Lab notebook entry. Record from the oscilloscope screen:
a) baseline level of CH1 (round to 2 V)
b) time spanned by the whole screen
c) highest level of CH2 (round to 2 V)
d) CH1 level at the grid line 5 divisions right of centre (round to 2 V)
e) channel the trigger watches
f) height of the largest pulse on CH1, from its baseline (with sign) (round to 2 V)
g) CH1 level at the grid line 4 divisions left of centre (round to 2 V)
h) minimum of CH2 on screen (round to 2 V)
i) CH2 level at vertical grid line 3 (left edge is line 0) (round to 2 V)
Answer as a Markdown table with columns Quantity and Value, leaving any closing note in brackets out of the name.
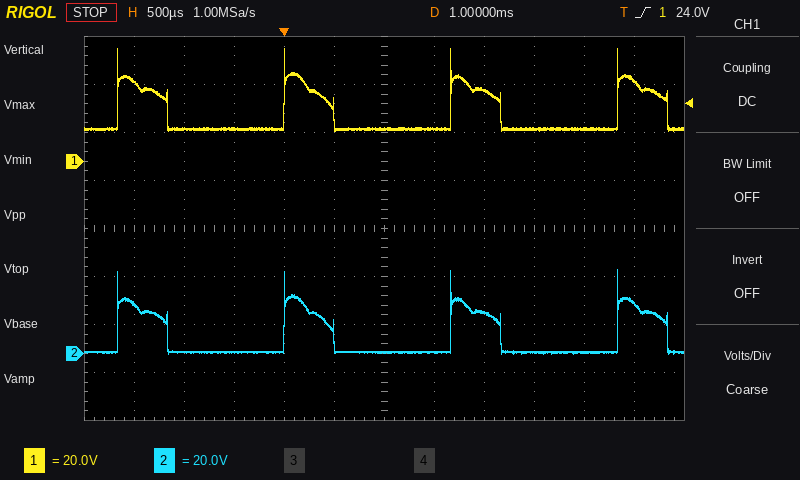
| Quantity | Value |
|---|---|
| baseline level of CH1 | 14 V |
| time spanned by the whole screen | 6 ms |
| highest level of CH2 | 34 V |
| CH1 level at the grid line 5 divisions right of centre | 34 V |
| channel the trigger watches | CH1 |
| height of the largest pulse on CH1, from its baseline (with sign) | +34 V |
| CH1 level at the grid line 4 divisions left of centre | 14 V |
| minimum of CH2 on screen | 0 V |
| CH2 level at vertical grid line 3 (left edge is line 0) | 0 V |
